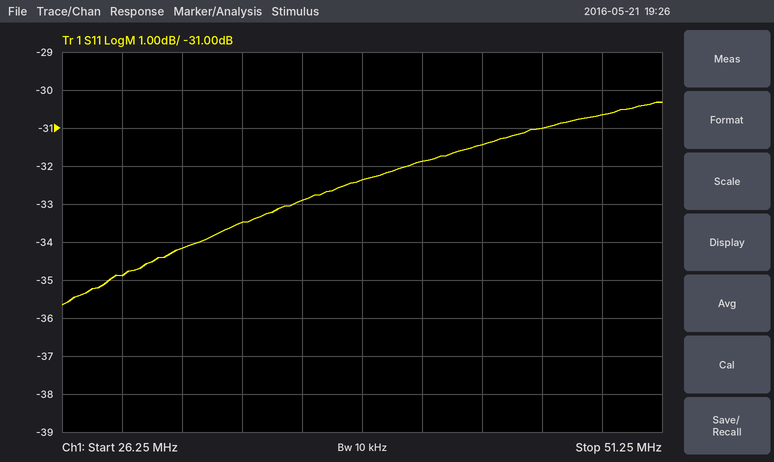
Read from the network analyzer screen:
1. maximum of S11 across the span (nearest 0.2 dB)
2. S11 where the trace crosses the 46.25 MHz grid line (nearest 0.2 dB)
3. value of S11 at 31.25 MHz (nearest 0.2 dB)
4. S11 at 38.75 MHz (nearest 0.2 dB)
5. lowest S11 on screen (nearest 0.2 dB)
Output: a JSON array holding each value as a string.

["-30.4 dB", "-31.0 dB", "-34.2 dB", "-32.4 dB", "-35.6 dB"]
